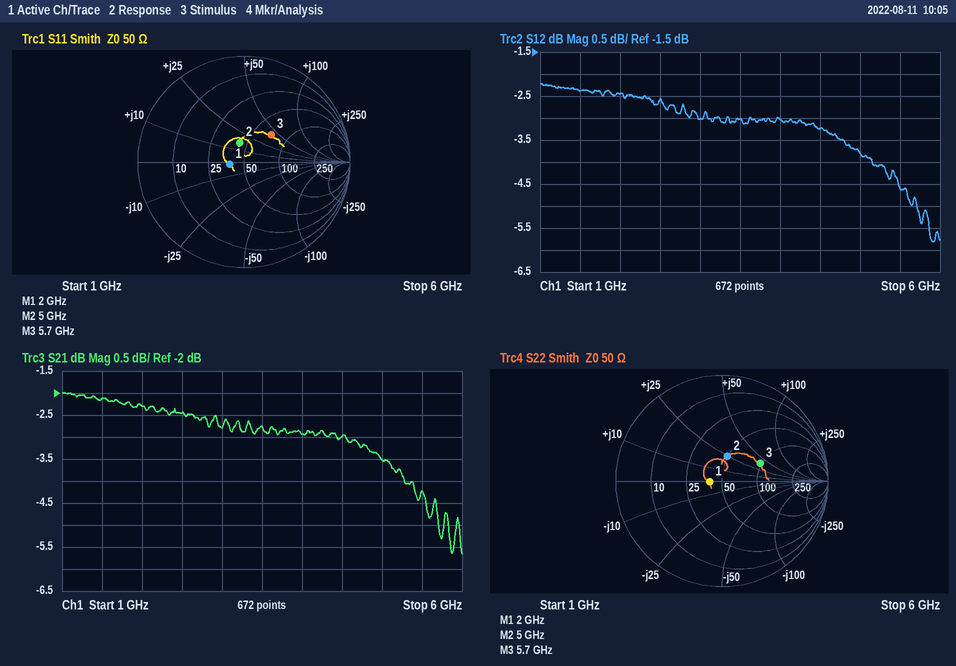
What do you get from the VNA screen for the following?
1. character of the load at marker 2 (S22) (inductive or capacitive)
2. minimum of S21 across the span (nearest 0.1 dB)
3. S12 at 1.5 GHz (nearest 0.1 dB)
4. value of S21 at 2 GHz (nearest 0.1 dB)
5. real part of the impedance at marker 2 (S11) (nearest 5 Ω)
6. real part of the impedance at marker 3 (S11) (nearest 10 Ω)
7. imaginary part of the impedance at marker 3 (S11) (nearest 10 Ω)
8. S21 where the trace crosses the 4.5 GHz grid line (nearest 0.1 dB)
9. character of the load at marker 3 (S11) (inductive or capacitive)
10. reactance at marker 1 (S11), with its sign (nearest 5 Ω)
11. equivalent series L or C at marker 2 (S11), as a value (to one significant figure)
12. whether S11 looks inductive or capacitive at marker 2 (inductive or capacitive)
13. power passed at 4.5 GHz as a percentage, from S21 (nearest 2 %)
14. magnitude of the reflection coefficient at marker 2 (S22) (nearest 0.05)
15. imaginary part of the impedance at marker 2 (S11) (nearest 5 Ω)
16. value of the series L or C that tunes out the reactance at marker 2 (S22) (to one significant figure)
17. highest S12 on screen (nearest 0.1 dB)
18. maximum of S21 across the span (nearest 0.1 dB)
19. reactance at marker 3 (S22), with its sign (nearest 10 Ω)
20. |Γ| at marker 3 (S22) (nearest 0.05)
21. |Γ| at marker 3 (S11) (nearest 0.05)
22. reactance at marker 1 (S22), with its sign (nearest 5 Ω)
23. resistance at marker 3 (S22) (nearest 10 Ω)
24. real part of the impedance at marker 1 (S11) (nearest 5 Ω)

inductive
-5.7 dB
-2.4 dB
-2.3 dB
45 Ω
70 Ω
+40 Ω
-3.0 dB
inductive
0 Ω
500 pH
inductive
50 %
0.25
+15 Ω
1 pF
-2.2 dB
-2.0 dB
+40 Ω
0.40
0.35
0 Ω
100 Ω
40 Ω
